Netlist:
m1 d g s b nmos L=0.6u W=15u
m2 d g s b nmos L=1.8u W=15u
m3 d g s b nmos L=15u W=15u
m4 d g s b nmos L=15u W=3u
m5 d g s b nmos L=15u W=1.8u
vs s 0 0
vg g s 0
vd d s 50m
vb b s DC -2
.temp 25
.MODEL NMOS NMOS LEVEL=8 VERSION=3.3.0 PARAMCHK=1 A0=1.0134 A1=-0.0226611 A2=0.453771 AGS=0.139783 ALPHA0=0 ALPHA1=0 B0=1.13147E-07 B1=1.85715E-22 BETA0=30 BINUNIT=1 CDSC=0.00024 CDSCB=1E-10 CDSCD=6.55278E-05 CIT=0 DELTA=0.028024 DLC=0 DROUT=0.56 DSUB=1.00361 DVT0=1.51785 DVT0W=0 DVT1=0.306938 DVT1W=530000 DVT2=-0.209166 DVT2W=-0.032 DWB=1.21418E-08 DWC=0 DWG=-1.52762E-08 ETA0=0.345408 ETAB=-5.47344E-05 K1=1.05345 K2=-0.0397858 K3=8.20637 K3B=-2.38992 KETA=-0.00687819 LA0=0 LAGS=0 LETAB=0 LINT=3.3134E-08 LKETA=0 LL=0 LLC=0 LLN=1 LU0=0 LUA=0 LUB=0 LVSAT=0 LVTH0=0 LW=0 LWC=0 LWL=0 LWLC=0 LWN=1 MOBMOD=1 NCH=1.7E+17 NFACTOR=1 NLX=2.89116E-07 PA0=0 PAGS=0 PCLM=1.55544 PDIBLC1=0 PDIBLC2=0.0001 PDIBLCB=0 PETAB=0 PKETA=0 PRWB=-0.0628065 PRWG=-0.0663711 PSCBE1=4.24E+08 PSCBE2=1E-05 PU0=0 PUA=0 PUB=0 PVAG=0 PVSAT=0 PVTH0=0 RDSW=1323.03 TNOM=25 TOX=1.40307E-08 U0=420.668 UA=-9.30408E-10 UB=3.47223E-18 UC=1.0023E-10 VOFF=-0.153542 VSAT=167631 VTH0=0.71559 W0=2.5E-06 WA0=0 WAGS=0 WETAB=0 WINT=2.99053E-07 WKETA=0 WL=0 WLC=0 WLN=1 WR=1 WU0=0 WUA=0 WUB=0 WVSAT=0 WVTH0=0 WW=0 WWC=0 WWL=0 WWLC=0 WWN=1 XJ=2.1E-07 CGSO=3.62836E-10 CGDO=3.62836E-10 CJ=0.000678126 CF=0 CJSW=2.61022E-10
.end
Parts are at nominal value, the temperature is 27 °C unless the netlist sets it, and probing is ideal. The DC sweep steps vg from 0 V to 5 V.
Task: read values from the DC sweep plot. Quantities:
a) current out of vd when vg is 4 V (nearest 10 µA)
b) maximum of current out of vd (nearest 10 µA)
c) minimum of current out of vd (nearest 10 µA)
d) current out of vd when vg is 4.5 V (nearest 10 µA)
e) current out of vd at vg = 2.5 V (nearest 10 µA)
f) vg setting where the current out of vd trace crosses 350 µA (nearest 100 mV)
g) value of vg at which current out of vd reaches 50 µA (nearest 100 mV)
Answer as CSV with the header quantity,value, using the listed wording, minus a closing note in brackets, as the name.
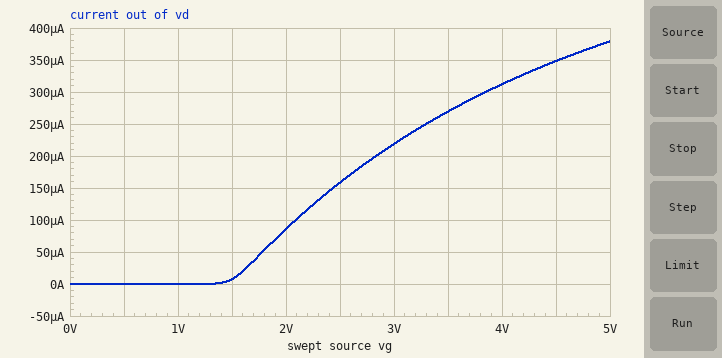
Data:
quantity,value
current out of vd when vg is 4 V,310 µA
maximum of current out of vd,380 µA
minimum of current out of vd,0 A
current out of vd when vg is 4.5 V,350 µA
current out of vd at vg = 2.5 V,160 µA
vg setting where the current out of vd trace crosses 350 µA,4.5 V
value of vg at which current out of vd reaches 50 µA,1.8 V
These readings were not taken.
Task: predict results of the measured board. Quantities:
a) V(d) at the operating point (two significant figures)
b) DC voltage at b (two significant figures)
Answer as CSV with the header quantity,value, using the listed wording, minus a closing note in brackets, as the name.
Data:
quantity,value
V(d) at the operating point,50 mV
DC voltage at b,-2.0 V
